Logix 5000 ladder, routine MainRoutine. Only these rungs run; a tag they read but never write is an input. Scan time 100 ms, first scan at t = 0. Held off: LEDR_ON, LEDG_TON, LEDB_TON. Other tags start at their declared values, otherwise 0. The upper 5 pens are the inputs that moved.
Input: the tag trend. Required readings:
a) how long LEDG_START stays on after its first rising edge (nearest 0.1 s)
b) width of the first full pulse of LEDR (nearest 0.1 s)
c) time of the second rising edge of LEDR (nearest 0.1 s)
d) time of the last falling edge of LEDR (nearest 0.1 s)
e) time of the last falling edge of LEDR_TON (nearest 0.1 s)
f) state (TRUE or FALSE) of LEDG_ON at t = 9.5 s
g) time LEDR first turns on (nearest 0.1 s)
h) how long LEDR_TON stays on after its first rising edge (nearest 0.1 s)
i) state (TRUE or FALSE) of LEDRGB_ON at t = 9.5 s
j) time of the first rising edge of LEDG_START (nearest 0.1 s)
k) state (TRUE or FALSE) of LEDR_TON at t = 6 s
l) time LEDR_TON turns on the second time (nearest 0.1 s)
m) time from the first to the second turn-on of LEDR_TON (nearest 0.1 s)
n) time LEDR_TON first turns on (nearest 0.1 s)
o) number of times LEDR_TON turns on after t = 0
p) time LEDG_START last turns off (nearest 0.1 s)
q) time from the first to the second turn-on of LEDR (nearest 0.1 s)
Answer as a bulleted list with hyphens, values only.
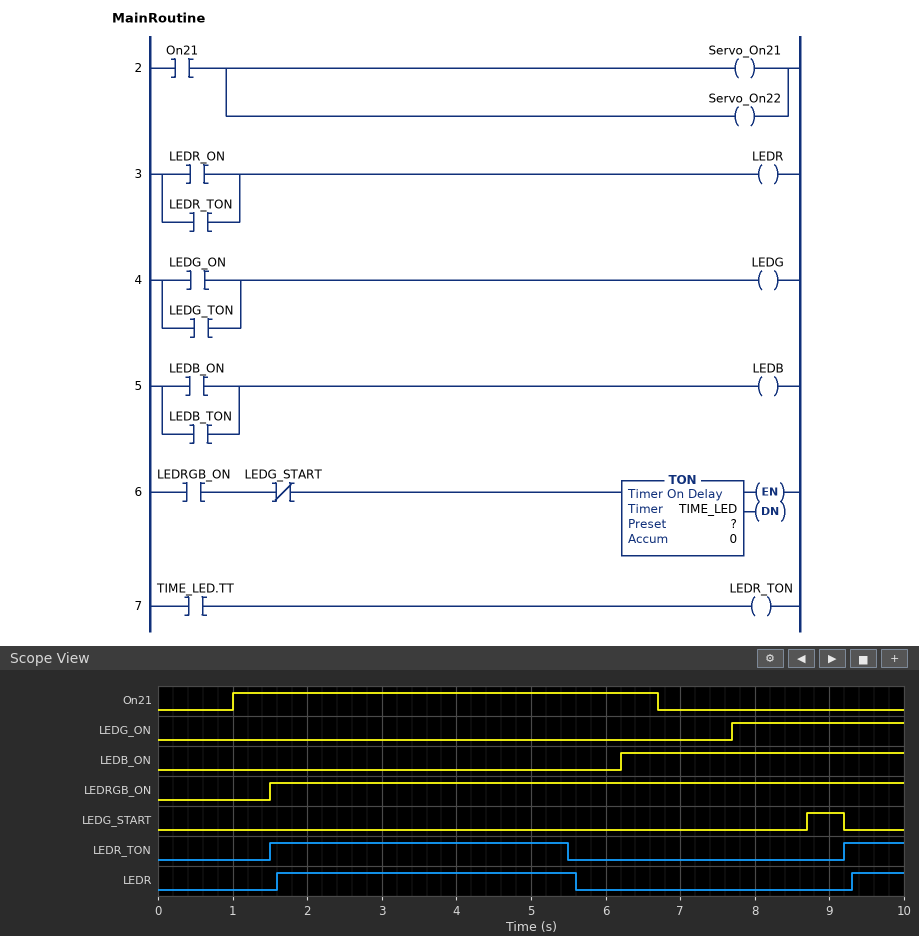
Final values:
- 0.5 s
- 4.0 s
- 9.3 s
- 5.6 s
- 5.5 s
- TRUE
- 1.6 s
- 4.0 s
- TRUE
- 8.7 s
- FALSE
- 9.2 s
- 7.7 s
- 1.5 s
- 2
- 9.2 s
- 7.7 s
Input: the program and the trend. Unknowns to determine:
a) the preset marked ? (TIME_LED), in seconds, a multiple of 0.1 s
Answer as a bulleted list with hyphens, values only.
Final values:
- 4.0 s
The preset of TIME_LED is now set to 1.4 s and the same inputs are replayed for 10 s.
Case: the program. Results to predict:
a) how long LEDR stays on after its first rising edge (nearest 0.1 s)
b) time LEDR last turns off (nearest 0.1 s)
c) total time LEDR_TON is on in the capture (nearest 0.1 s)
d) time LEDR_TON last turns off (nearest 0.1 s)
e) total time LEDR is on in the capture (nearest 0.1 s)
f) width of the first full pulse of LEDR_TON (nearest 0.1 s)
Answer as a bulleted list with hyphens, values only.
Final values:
- 1.4 s
- 3.0 s
- 2.2 s
- 2.9 s
- 2.1 s
- 1.4 s
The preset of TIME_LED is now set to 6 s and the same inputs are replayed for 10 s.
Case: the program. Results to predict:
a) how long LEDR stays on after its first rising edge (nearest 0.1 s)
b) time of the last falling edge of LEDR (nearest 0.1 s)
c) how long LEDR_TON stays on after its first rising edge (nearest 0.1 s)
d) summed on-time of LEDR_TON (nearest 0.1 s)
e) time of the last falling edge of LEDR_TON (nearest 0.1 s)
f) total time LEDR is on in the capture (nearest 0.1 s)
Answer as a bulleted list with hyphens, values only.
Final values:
- 6.0 s
- 7.6 s
- 6.0 s
- 6.8 s
- 7.5 s
- 6.7 s
